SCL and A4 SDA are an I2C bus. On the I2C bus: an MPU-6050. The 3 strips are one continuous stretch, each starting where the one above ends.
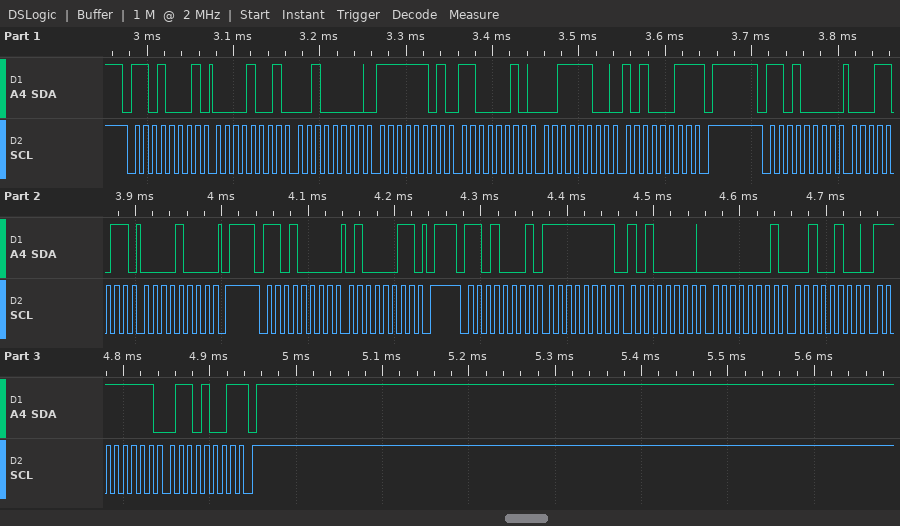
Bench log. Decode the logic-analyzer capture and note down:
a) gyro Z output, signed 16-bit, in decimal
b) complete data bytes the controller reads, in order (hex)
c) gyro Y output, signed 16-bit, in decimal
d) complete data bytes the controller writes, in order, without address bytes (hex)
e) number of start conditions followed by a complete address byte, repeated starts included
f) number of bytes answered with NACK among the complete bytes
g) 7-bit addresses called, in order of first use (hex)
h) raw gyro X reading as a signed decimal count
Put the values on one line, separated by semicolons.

-151; 09 20 FD C2 3C A3 FF A0 01 24 FF 69; 292; 1B 08 43; 4; 2; 0x68; -96
